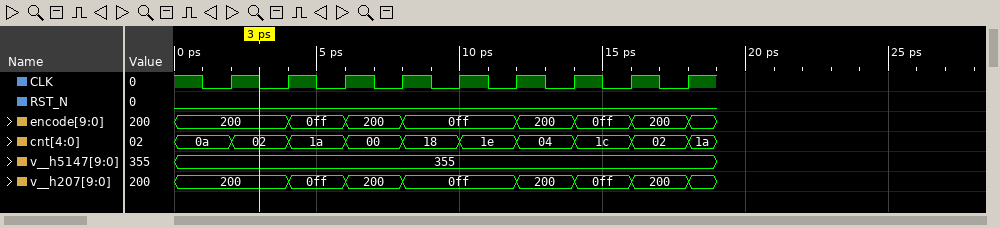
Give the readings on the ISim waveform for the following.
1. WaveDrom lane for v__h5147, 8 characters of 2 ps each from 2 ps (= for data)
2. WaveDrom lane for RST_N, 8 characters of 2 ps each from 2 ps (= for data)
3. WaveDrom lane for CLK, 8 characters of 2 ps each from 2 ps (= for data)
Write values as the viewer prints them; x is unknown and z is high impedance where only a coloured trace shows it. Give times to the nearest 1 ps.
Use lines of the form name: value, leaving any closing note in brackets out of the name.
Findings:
WaveDrom lane for v__h5147, 8 characters of 2 ps each from 2 ps: {name: 'v__h5147', wave: '=.......', data: '355'}
WaveDrom lane for RST_N, 8 characters of 2 ps each from 2 ps: {name: 'RST_N', wave: '0.......'}
WaveDrom lane for CLK, 8 characters of 2 ps each from 2 ps: {name: 'CLK', wave: 'p.......'}
